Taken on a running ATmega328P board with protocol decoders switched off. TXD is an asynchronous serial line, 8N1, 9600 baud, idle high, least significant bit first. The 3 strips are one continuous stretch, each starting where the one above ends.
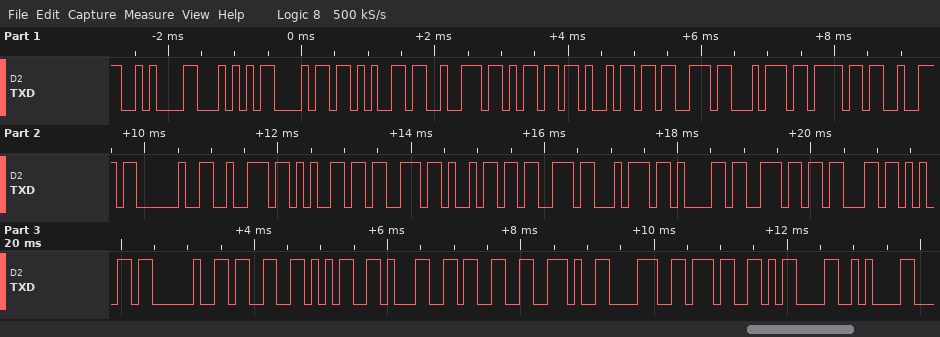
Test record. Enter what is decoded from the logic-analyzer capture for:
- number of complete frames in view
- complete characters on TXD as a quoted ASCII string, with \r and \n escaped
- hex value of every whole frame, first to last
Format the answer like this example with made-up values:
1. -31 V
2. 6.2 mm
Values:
1. 32
2. "\nThermistor resistance 3513.87\r\n"
3. 0A 54 68 65 72 6D 69 73 74 6F 72 20 72 65 73 69 73 74 61 6E 63 65 20 33 35 31 33 2E 38 37 0D 0A
